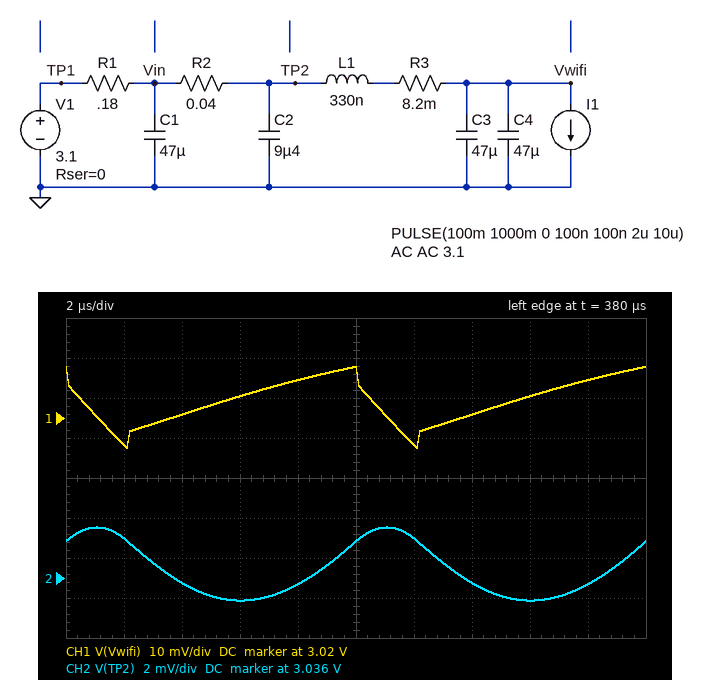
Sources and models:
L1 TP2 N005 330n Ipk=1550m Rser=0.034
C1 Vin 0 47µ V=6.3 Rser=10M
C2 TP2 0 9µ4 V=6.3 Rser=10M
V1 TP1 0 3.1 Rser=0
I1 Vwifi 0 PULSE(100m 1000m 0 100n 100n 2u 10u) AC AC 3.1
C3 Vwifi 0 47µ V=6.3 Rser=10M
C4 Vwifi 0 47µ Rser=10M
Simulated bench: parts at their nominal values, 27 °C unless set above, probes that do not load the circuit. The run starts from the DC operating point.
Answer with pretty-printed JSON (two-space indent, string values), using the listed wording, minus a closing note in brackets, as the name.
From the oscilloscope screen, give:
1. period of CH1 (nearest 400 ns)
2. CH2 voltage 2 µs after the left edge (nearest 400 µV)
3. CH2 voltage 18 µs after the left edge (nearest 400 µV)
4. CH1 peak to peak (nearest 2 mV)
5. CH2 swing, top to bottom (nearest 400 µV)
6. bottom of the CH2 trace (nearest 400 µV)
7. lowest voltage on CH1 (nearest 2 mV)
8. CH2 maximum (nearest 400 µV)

{
  "period of CH1": "10.0 µs",
  "CH2 voltage 2 µs after the left edge": "3.0380 V",
  "CH2 voltage 18 µs after the left edge": "3.0356 V",
  "CH1 peak to peak": "20 mV",
  "CH2 swing, top to bottom": "3.6 mV",
  "bottom of the CH2 trace": "3.0348 V",
  "lowest voltage on CH1": "3.012 V",
  "CH2 maximum": "3.0384 V"
}
